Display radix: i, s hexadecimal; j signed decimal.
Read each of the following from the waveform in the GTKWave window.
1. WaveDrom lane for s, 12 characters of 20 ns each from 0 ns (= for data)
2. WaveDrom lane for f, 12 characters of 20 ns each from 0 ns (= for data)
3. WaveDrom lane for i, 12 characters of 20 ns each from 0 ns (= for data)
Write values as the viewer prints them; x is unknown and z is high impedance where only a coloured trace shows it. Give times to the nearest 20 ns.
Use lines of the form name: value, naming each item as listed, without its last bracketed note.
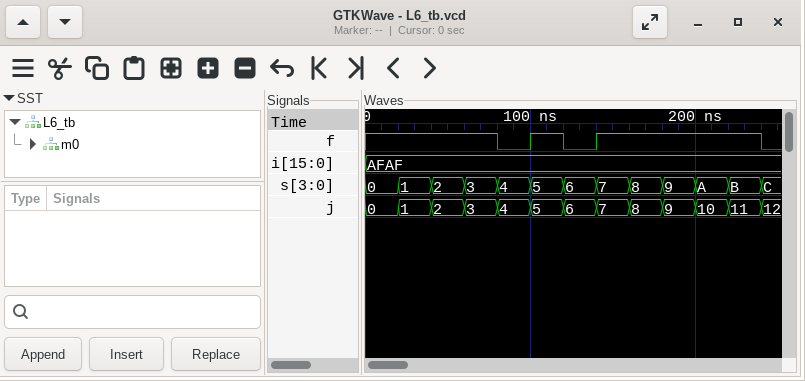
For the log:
WaveDrom lane for s, 12 characters of 20 ns each from 0 ns: {name: 's', wave: '============', data: '0 1 2 3 4 5 6 7 8 9 A B'}
WaveDrom lane for f, 12 characters of 20 ns each from 0 ns: {name: 'f', wave: '1...0101....'}
WaveDrom lane for i, 12 characters of 20 ns each from 0 ns: {name: 'i', wave: '=...........', data: 'AFAF'}
